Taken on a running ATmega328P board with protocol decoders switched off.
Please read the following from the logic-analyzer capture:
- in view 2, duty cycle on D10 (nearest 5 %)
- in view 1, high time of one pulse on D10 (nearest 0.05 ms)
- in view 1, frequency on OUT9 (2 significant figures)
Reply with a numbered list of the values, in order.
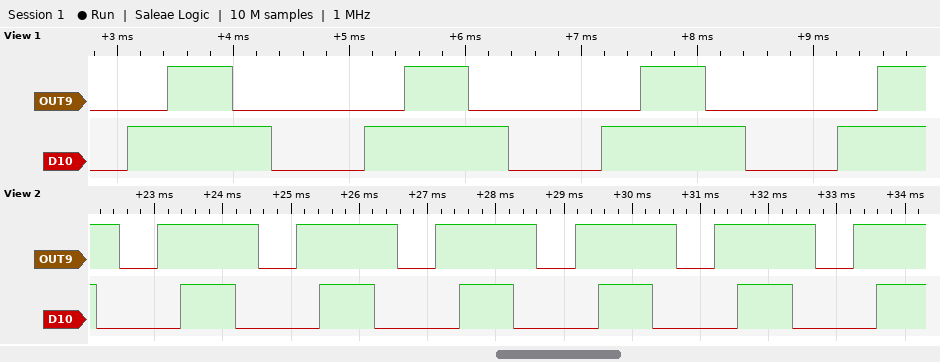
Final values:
1. 40 %
2. 1.25 ms
3. 490 Hz
